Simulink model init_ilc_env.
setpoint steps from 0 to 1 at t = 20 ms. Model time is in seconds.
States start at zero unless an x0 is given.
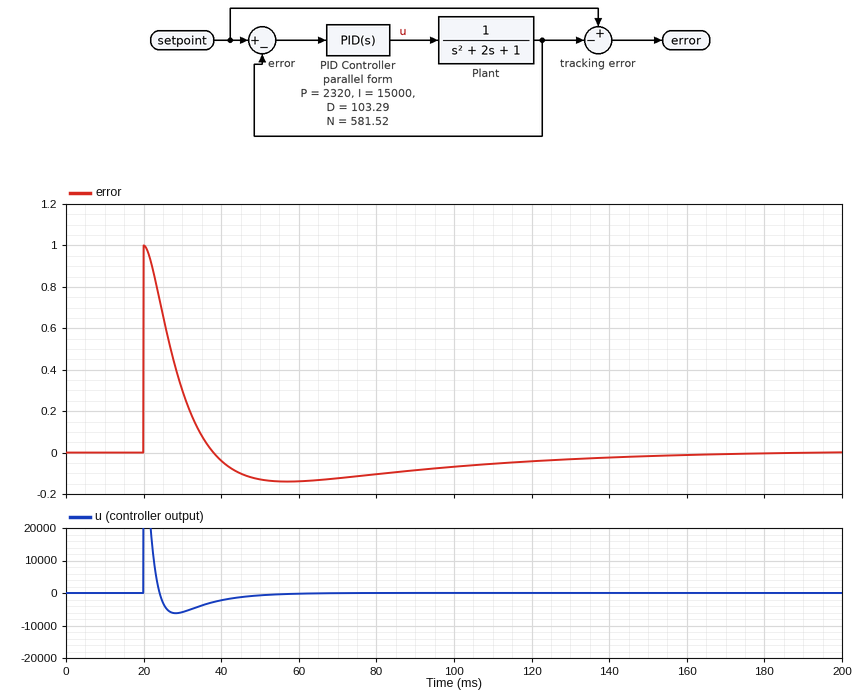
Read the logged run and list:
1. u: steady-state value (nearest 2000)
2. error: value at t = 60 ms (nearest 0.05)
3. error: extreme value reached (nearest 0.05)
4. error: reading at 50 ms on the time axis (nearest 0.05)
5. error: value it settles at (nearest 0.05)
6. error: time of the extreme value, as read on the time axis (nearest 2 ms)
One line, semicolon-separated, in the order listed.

0; -0.15; 1.00; -0.15; 0.00; 20 ms
